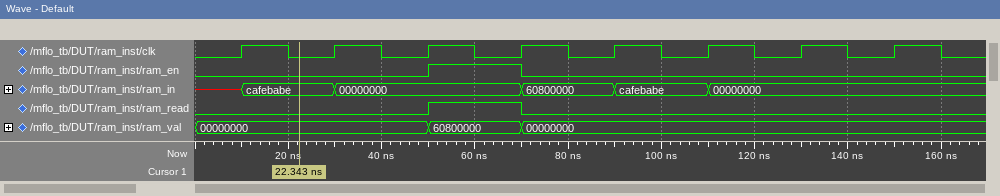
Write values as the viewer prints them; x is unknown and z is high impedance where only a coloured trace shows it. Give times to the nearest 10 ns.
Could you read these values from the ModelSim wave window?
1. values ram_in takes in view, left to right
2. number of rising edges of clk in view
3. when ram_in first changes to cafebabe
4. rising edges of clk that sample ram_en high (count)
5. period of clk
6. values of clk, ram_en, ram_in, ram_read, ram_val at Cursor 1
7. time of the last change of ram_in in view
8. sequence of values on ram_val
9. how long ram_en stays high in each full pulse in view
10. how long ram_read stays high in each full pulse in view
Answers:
x, cafebabe, 00000000, 60800000, cafebabe, 00000000
8
10 ns
1
20 ns
clk=0, ram_en=0, ram_in=cafebabe, ram_read=0, ram_val=00000000
110 ns
00000000, 60800000, 00000000
20 ns
20 ns
